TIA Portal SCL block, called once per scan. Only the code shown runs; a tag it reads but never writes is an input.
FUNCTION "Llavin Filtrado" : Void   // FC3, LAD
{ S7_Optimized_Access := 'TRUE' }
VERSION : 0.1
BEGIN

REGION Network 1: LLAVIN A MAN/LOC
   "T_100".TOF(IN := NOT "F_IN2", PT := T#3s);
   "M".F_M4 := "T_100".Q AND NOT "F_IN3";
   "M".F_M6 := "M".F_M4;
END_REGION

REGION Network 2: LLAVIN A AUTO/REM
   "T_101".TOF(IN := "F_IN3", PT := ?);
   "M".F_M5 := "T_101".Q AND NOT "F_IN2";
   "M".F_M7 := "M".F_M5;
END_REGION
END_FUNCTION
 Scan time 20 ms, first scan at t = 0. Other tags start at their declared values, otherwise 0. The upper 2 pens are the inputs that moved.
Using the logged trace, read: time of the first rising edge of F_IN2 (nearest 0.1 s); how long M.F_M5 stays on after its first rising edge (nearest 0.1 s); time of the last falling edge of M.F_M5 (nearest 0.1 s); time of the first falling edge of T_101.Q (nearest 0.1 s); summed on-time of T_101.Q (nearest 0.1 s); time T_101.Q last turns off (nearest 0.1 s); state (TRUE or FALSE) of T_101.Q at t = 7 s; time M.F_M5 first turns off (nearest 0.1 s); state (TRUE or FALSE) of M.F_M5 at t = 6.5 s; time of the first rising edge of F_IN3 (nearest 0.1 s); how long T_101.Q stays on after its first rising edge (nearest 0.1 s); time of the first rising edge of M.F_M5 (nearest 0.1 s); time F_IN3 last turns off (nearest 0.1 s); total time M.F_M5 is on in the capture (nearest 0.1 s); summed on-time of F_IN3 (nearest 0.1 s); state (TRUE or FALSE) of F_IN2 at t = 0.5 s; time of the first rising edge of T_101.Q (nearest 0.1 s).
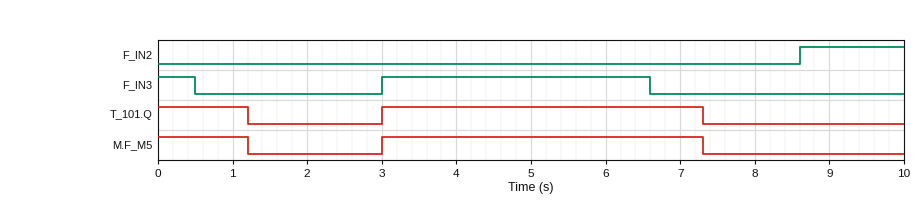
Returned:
8.6 s
4.3 s
7.3 s
1.2 s
5.5 s
7.3 s
TRUE
1.2 s
TRUE
3.0 s
4.3 s
3.0 s
6.6 s
5.5 s
4.1 s
FALSE
3.0 s
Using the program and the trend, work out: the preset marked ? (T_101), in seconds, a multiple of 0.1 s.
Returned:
0.7 s
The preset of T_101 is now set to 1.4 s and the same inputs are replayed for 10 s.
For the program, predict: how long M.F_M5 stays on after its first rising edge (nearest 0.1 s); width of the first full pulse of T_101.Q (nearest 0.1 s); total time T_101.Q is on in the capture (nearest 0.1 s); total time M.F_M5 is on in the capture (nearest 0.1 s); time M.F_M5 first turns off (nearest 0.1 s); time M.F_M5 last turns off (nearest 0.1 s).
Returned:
5.0 s
5.0 s
6.9 s
6.9 s
1.9 s
8.0 s
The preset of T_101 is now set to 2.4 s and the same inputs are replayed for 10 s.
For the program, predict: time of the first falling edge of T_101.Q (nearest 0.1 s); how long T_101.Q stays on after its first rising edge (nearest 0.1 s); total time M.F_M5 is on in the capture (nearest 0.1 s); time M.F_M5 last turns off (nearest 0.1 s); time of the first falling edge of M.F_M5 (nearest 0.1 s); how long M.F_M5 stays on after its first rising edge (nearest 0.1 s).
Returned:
2.9 s
6.0 s
8.5 s
8.6 s
2.9 s
5.6 s
